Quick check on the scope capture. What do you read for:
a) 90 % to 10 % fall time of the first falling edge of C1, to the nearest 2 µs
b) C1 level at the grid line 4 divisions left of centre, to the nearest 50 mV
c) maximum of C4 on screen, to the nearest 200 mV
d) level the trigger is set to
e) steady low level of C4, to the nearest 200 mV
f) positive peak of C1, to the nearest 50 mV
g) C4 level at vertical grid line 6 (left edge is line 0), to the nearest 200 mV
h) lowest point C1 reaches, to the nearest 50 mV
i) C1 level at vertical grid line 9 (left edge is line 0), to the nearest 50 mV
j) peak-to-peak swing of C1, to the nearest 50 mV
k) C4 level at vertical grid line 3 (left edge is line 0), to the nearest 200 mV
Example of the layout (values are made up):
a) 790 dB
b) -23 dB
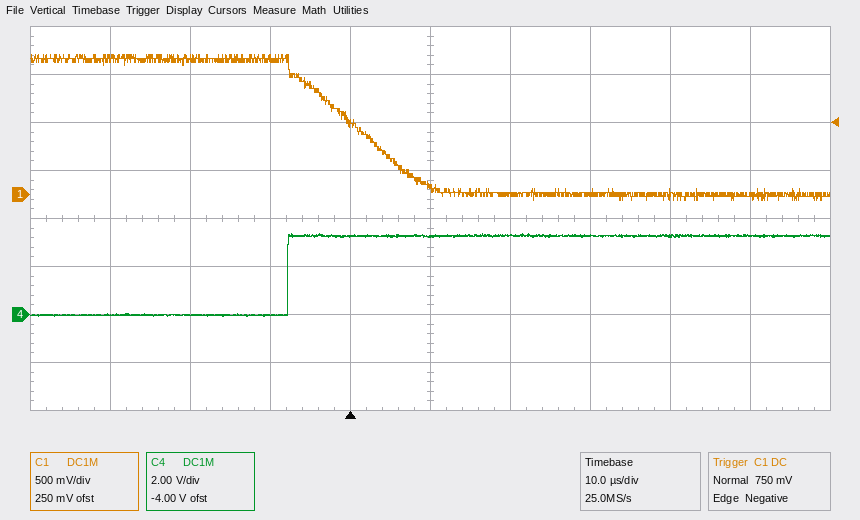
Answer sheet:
a) 16 µs
b) 1.40 V
c) 3.4 V
d) 750 mV
e) 0.0 V
f) 1.45 V
g) 3.2 V
h) -50 mV
i) 0 mV
j) 1.50 V
k) 0.0 V
